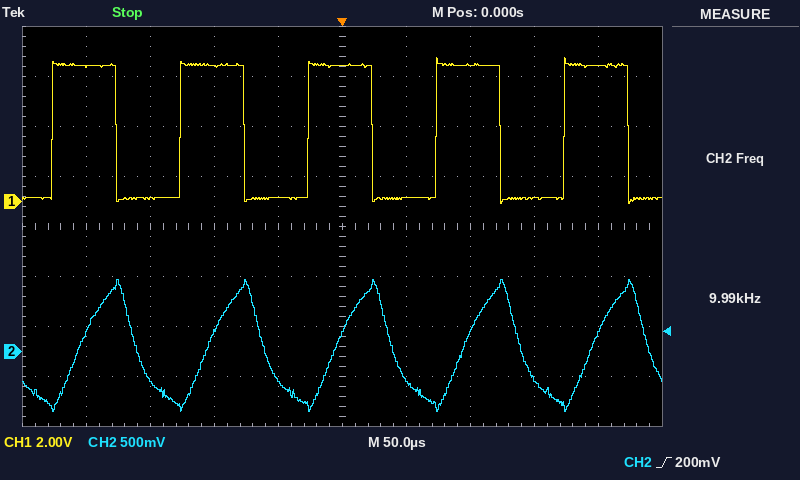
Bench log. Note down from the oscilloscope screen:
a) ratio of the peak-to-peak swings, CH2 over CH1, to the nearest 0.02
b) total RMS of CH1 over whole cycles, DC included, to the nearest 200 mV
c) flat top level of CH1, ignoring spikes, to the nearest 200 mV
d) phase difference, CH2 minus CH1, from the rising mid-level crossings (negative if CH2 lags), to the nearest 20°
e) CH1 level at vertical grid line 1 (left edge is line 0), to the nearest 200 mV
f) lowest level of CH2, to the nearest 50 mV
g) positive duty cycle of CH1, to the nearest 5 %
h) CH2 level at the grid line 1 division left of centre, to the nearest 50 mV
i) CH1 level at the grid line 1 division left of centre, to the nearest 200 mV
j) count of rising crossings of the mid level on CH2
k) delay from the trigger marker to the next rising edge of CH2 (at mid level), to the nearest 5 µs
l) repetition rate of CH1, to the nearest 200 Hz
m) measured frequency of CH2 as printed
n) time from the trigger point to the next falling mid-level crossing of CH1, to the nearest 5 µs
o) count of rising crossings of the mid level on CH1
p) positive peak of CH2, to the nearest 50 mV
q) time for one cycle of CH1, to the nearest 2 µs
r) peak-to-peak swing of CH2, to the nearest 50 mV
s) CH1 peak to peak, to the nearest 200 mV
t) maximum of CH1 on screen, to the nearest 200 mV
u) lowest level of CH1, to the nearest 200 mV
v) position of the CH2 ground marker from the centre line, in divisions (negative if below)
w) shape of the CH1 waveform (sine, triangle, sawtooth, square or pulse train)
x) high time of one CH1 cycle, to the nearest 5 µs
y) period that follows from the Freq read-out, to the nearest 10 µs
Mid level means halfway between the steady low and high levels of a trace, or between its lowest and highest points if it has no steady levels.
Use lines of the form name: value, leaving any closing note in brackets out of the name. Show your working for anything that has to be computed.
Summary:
ratio of the peak-to-peak swings, CH2 over CH1, to the nearest 0.02: 1.30 V / 5.8 V ≈ 0.22
total RMS of CH1 over whole cycles, DC included, to the nearest 200 mV: √(0.5 × (5.4 V)² + 0.5 × (0.0 V)²) ≈ 3.8 V
flat top level of CH1, ignoring spikes, to the nearest 200 mV: 5.4 V
phase difference, CH2 minus CH1, from the rising mid-level crossings (negative if CH2 lags), to the nearest 20°: -80°
CH1 level at vertical grid line 1 (left edge is line 0), to the nearest 200 mV: 5.4 V
lowest level of CH2, to the nearest 50 mV: -600 mV
positive duty cycle of CH1, to the nearest 5 %: 50 µs / 100 µs ≈ 50 %
CH2 level at the grid line 1 division left of centre, to the nearest 50 mV: -300 mV
CH1 level at the grid line 1 division left of centre, to the nearest 200 mV: 200 mV
count of rising crossings of the mid level on CH2: 5
delay from the trigger marker to the next rising edge of CH2 (at mid level), to the nearest 5 µs: 95 µs
repetition rate of CH1, to the nearest 200 Hz: 1 / 100 µs ≈ 10.0 kHz
measured frequency of CH2 as printed: 9.99 kHz
time from the trigger point to the next falling mid-level crossing of CH1, to the nearest 5 µs: 25 µs
count of rising crossings of the mid level on CH1: 5
positive peak of CH2, to the nearest 50 mV: 700 mV
time for one cycle of CH1, to the nearest 2 µs: 100 µs
peak-to-peak swing of CH2, to the nearest 50 mV: 700 mV − (-600 mV) = 1.30 V
CH1 peak to peak, to the nearest 200 mV: 5.8 V − (0.0 V) = 5.8 V
maximum of CH1 on screen, to the nearest 200 mV: 5.8 V
lowest level of CH1, to the nearest 200 mV: 0.0 V
position of the CH2 ground marker from the centre line, in divisions: -2.5 div
shape of the CH1 waveform: square
high time of one CH1 cycle, to the nearest 5 µs: 50 µs
period that follows from the Freq read-out, to the nearest 10 µs: 1 / 9.99 kHz ≈ 100 µs
